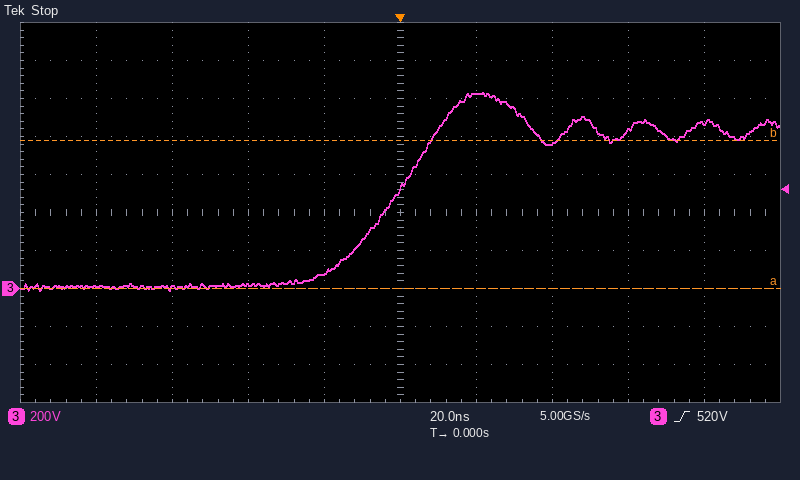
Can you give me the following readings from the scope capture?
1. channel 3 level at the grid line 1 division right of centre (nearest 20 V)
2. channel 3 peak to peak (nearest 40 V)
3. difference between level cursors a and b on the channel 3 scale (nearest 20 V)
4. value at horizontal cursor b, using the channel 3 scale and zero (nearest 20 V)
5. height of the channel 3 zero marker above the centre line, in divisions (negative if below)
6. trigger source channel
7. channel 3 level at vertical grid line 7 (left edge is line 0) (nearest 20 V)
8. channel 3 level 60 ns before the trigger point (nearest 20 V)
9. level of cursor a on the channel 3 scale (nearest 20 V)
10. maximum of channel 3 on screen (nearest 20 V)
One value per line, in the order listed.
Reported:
1.02 kV
1.04 kV
780 V
780 V
-2.0 div
channel 3
760 V
0 V
0 V
1.04 kV
